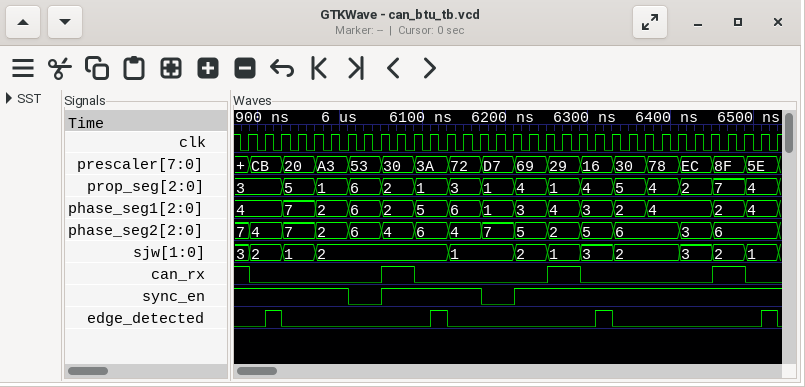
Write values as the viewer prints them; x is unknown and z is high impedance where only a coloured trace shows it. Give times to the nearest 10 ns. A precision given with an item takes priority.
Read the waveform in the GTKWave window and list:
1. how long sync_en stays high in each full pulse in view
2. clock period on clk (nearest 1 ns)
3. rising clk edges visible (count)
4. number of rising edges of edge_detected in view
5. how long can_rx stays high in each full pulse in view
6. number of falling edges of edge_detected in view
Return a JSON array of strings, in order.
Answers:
["120 ns", "20 ns", "33", "4", "40 ns, 40 ns, 40 ns", "4"]
